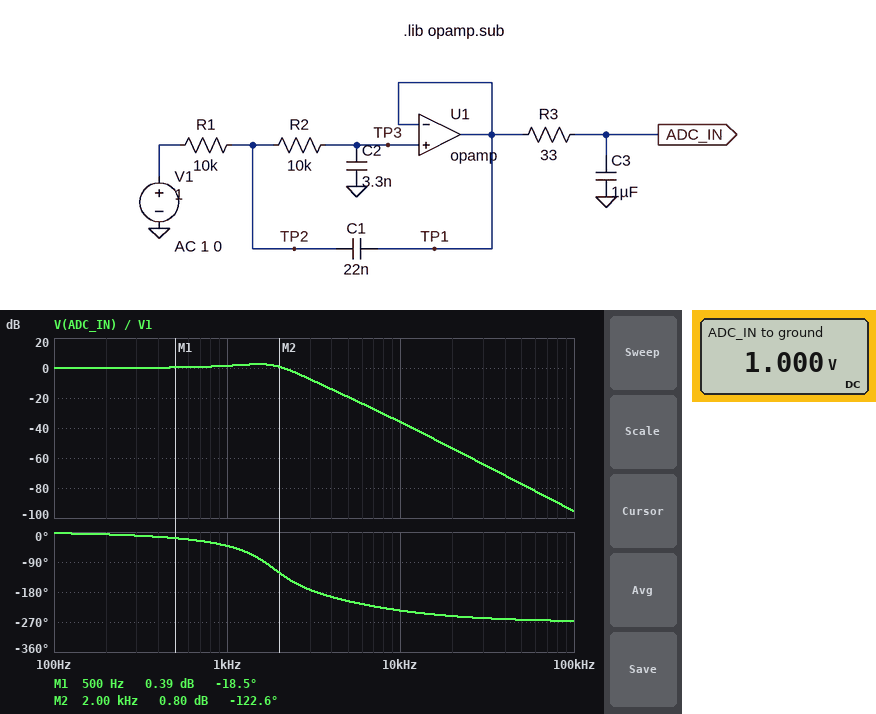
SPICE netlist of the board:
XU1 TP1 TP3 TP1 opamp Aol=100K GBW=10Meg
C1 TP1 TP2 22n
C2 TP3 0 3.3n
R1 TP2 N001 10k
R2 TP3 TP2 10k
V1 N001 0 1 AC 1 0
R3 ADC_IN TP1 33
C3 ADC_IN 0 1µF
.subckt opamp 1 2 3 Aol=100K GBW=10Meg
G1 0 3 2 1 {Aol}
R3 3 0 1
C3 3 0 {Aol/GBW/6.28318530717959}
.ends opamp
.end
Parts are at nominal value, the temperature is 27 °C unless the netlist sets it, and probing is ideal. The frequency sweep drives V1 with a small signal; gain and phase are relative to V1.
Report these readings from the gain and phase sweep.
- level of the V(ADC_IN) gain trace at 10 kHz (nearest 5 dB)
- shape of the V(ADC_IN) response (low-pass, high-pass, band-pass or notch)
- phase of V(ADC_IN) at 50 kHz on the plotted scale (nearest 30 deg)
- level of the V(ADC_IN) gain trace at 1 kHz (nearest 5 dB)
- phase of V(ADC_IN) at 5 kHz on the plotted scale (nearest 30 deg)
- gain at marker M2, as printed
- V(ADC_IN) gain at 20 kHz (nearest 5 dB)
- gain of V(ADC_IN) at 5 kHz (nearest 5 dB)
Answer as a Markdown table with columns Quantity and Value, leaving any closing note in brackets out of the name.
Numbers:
| Quantity | Value |
|---|---|
| level of the V(ADC_IN) gain trace at 10 kHz | -35 dB |
| shape of the V(ADC_IN) response | low-pass |
| phase of V(ADC_IN) at 50 kHz on the plotted scale | -270 deg |
| level of the V(ADC_IN) gain trace at 1 kHz | 0 dB |
| phase of V(ADC_IN) at 5 kHz on the plotted scale | -210 deg |
| gain at marker M2, as printed | 0.80 dB |
| V(ADC_IN) gain at 20 kHz | -55 dB |
| gain of V(ADC_IN) at 5 kHz | -20 dB |
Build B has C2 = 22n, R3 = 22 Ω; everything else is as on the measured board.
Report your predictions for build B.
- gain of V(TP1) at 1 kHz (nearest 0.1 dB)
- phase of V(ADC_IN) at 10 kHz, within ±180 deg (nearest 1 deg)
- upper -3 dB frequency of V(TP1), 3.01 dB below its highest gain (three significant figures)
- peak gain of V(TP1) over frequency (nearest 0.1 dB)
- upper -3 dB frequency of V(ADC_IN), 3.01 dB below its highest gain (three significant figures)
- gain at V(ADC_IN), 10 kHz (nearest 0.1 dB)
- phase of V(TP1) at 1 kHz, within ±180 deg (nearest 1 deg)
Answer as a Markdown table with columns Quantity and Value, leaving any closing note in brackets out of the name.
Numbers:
| Quantity | Value |
|---|---|
| gain of V(TP1) at 1 kHz | -9.3 dB |
| phase of V(ADC_IN) at 10 kHz, within ±180 deg | 134 deg |
| upper -3 dB frequency of V(TP1), 3.01 dB below its highest gain | 466 Hz |
| peak gain of V(TP1) over frequency | 0 dB |
| upper -3 dB frequency of V(ADC_IN), 3.01 dB below its highest gain | 464 Hz |
| gain at V(ADC_IN), 10 kHz | -50.3 dB |
| phase of V(TP1) at 1 kHz, within ±180 deg | -108 deg |
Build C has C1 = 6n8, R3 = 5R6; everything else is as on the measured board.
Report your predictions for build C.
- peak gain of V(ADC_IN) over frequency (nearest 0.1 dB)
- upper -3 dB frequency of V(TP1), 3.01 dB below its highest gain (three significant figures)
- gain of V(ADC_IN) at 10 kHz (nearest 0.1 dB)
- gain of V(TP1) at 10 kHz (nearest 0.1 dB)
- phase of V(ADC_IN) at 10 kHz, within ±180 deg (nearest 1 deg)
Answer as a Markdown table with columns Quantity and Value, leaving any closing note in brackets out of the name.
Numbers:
| Quantity | Value |
|---|---|
| peak gain of V(ADC_IN) over frequency | 0 dB |
| upper -3 dB frequency of V(TP1), 3.01 dB below its highest gain | 3.41 kHz |
| gain of V(ADC_IN) at 10 kHz | -19.5 dB |
| gain of V(TP1) at 10 kHz | -19.0 dB |
| phase of V(ADC_IN) at 10 kHz, within ±180 deg | -172 deg |
